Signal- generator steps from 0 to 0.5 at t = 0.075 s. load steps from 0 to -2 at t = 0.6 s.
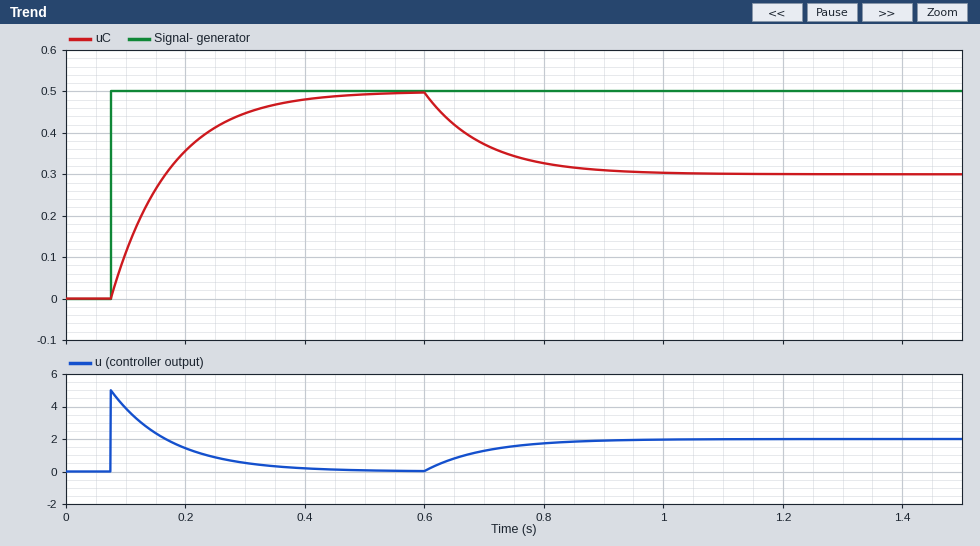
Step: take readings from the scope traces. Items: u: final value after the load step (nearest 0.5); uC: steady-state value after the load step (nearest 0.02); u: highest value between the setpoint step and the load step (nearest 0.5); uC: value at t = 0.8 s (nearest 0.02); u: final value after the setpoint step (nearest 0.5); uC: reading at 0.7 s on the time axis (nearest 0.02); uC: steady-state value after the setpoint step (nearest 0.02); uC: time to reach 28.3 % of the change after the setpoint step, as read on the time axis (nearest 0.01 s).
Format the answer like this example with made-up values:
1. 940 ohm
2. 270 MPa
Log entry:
1. 2.0
2. 0.30
3. 5.0
4. 0.32
5. 0.0
6. 0.38
7. 0.50
8. 0.11 s
